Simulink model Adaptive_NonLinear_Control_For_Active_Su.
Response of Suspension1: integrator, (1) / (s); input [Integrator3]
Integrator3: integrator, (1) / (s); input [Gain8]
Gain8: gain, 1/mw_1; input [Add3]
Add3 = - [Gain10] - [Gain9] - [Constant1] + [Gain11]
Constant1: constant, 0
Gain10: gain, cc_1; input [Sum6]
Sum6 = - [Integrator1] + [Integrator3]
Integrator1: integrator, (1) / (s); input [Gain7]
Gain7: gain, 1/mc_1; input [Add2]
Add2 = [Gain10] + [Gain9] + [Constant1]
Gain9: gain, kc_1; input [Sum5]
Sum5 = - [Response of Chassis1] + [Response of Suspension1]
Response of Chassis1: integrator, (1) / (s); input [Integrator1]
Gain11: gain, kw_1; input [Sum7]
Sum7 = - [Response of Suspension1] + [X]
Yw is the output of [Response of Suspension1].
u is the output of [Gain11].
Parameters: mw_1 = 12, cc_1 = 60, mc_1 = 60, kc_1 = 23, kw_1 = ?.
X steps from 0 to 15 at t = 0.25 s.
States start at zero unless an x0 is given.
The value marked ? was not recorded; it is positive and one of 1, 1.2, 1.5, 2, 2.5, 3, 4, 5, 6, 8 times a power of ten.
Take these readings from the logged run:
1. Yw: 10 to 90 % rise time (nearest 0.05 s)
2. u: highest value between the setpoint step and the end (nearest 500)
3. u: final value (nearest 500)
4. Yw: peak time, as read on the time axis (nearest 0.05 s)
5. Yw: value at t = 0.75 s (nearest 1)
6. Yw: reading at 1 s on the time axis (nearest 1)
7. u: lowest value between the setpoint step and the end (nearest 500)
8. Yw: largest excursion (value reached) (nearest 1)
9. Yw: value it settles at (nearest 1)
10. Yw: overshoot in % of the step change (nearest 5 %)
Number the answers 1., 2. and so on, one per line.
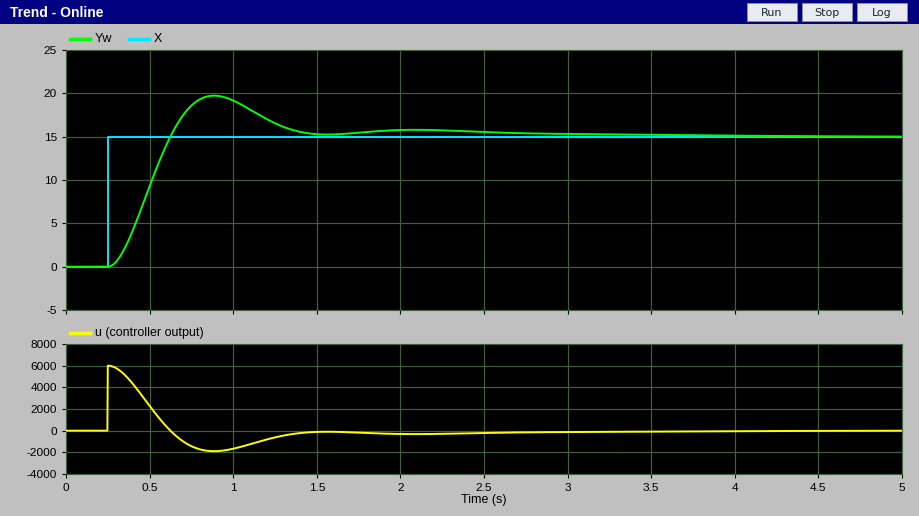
1. 0.25 s
2. 6000
3. 0
4. 0.90 s
5. 19
6. 19
7. -2000
8. 20
9. 15
10. 30 %
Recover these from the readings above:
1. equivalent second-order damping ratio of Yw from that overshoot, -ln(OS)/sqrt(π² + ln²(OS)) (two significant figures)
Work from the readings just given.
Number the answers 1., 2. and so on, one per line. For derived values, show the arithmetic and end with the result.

1. ln(0.3) = -1.204; 1.204 / sqrt(9.870 + 1.450) = 0.36
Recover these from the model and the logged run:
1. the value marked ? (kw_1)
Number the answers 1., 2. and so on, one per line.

1. 400
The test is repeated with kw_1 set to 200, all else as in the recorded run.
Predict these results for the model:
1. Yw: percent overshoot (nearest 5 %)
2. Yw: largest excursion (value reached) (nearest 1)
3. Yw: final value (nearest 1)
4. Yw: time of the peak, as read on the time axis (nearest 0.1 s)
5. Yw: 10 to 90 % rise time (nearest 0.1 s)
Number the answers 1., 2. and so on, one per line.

1. 25 %
2. 19
3. 15
4. 1.3 s
5. 0.4 s
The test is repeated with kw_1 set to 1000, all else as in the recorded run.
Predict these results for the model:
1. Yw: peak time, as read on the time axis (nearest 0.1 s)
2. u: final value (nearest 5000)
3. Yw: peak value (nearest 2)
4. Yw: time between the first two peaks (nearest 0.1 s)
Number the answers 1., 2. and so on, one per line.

1. 0.6 s
2. 0
3. 22
4. 0.7 s
